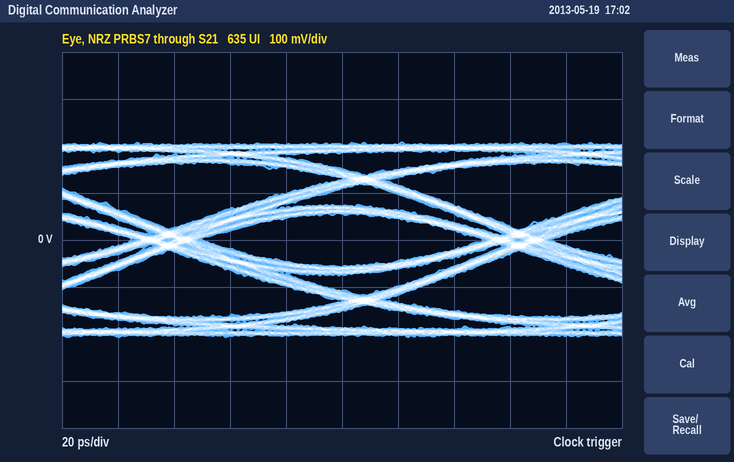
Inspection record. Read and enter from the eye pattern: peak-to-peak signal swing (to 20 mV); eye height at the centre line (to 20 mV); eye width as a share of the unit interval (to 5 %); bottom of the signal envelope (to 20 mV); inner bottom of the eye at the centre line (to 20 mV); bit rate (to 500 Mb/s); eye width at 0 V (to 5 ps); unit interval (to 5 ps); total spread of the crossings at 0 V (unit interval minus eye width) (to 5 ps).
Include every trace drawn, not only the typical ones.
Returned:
420 mV
120 mV
80 %
-200 mV
-60 mV
8.0 Gb/s
100 ps
125 ps
25 ps
